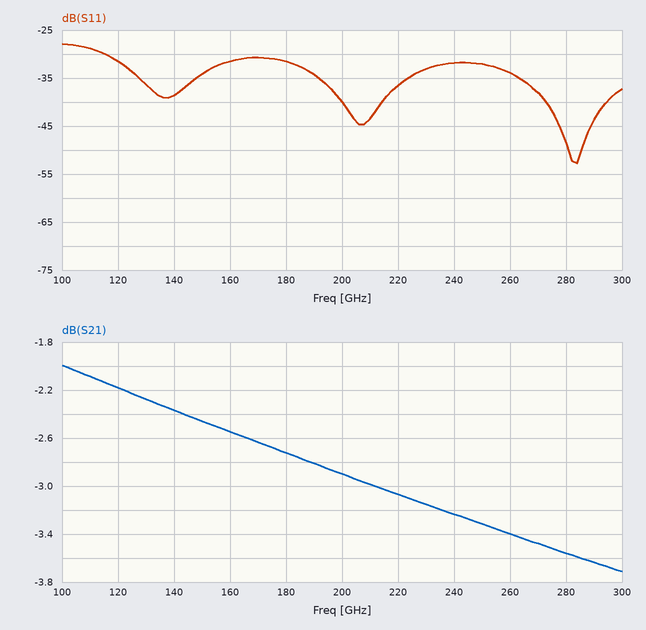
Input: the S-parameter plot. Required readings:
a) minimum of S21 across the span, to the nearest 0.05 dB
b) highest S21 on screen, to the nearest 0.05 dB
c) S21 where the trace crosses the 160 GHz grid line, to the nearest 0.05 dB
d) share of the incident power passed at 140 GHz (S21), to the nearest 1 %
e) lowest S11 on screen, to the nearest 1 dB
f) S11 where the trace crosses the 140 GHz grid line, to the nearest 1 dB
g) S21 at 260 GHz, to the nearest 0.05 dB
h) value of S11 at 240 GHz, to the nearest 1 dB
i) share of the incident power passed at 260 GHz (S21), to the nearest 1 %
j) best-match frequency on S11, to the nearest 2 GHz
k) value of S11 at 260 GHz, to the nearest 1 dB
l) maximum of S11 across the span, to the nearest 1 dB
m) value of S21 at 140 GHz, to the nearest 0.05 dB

-3.70 dB
-2.00 dB
-2.55 dB
58 %
-53 dB
-39 dB
-3.40 dB
-32 dB
46 %
284 GHz
-34 dB
-28 dB
-2.35 dB
